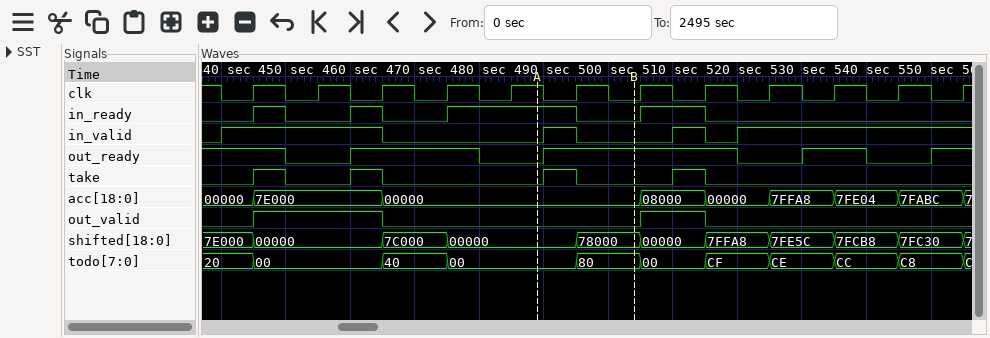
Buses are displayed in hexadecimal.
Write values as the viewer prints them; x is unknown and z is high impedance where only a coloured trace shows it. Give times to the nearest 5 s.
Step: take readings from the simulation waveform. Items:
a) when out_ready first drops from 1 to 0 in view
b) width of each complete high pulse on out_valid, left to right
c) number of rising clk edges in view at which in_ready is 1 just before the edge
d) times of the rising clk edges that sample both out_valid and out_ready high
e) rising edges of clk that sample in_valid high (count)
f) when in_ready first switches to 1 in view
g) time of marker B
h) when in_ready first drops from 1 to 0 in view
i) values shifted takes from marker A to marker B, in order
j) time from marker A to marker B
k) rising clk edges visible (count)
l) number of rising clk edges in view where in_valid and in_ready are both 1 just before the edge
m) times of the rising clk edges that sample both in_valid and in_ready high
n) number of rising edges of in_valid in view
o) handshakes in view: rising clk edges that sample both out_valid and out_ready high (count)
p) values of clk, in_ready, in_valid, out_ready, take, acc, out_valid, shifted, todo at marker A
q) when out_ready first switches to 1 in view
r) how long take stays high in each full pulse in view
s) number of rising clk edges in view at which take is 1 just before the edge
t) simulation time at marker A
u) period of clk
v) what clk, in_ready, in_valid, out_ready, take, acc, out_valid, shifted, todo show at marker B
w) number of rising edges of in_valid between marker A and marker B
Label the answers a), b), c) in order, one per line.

a) 450 s
b) 20 s, 10 s
c) 4
d) 465 s, 515 s
e) 9
f) 445 s
g) 505 s
h) 450 s
i) 00000, 78000
j) 15 s
k) 12
l) 3
m) 465 s, 495 s, 515 s
n) 4
o) 2
p) clk=1, in_ready=1, in_valid=0, out_ready=0, take=0, acc=00000, out_valid=0, shifted=00000, todo=00
q) 460 s
r) 5 s, 5 s, 5 s, 5 s
s) 3
t) 490 s
u) 10 s
v) clk=0, in_ready=0, in_valid=0, out_ready=1, take=0, acc=00000, out_valid=0, shifted=78000, todo=80
w) 1
